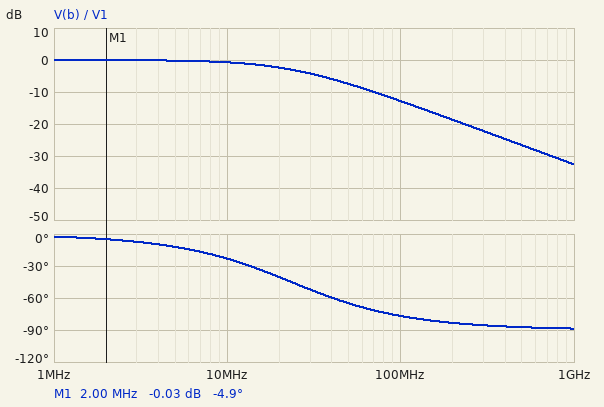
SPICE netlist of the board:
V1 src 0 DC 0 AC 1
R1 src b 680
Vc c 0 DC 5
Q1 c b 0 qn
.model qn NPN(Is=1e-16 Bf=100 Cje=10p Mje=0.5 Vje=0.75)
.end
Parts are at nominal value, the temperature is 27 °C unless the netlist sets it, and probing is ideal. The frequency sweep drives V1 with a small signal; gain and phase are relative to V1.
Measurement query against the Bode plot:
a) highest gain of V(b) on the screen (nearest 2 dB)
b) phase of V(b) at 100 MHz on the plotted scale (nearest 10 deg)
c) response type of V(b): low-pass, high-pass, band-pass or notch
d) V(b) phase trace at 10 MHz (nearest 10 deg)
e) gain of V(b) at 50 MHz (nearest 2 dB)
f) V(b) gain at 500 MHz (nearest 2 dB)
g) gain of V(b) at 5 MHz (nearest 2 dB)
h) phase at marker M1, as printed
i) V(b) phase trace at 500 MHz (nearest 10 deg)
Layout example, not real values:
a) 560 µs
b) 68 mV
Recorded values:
a) 0 dB
b) -80 deg
c) low-pass
d) -20 deg
e) -8 dB
f) -26 dB
g) 0 dB
h) -4.9 deg
i) -90 deg
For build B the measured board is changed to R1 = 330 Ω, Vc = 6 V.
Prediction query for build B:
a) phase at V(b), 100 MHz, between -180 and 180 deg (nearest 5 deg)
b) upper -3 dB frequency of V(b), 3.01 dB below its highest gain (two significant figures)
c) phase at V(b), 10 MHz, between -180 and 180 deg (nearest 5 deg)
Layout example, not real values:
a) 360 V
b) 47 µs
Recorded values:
a) -65 deg
b) 48 MHz
c) -10 deg
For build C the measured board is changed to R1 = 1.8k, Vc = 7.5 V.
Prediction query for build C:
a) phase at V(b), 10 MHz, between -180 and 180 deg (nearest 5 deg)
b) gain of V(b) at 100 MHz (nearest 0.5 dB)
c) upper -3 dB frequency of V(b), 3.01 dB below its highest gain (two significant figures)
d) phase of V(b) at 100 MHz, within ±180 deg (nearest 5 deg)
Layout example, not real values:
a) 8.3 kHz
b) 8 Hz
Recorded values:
a) -50 deg
b) -21.0 dB
c) 8.8 MHz
d) -85 deg
